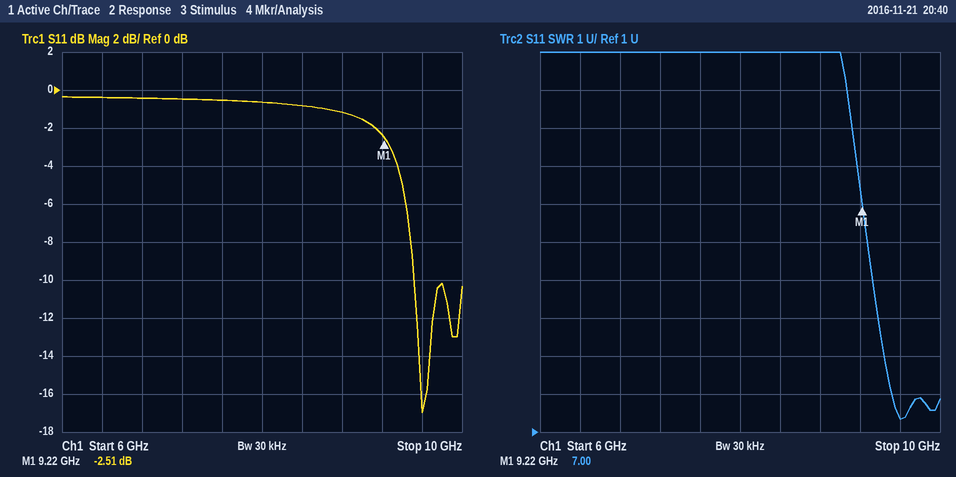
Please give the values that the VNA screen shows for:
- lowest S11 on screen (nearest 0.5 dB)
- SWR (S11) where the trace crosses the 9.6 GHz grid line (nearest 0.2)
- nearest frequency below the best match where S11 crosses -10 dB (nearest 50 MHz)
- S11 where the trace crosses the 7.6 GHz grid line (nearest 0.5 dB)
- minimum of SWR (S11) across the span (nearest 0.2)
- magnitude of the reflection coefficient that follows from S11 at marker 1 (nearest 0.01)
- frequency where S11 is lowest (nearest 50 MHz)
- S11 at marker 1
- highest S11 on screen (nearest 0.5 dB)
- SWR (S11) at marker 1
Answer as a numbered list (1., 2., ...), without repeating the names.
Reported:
1. -17.0 dB
2. 1.4
3. 9.50 GHz
4. -0.5 dB
5. 1.4
6. 0.75
7. 9.60 GHz
8. -2.51 dB
9. -0.5 dB
10. 7.00
